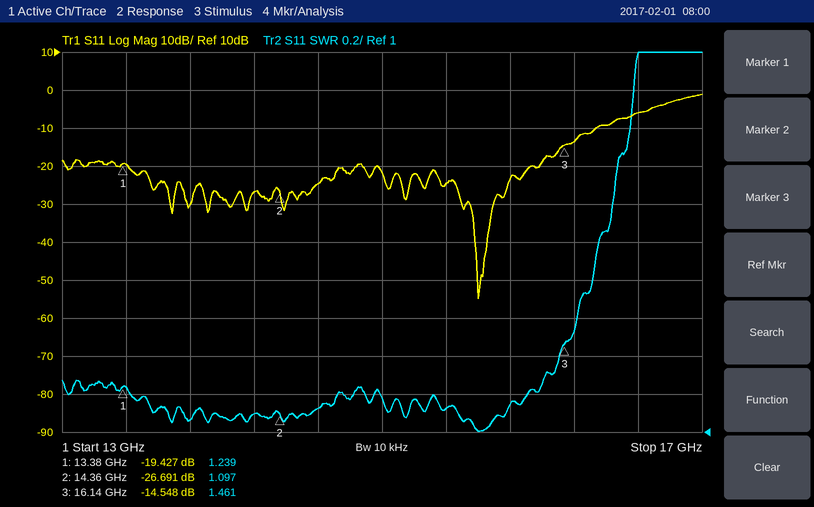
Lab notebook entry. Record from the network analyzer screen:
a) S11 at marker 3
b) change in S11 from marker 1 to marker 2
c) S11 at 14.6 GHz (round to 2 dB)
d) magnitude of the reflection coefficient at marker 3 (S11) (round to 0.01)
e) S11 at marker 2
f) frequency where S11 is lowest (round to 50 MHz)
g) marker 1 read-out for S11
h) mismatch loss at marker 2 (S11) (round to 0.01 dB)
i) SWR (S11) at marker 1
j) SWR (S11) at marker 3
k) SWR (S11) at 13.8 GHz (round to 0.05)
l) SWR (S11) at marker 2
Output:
-14.548 dB
-7.264 dB
-24 dB
0.19
-26.691 dB
15.60 GHz
-19.427 dB
0.01 dB
1.239
1.461
1.05
1.097
